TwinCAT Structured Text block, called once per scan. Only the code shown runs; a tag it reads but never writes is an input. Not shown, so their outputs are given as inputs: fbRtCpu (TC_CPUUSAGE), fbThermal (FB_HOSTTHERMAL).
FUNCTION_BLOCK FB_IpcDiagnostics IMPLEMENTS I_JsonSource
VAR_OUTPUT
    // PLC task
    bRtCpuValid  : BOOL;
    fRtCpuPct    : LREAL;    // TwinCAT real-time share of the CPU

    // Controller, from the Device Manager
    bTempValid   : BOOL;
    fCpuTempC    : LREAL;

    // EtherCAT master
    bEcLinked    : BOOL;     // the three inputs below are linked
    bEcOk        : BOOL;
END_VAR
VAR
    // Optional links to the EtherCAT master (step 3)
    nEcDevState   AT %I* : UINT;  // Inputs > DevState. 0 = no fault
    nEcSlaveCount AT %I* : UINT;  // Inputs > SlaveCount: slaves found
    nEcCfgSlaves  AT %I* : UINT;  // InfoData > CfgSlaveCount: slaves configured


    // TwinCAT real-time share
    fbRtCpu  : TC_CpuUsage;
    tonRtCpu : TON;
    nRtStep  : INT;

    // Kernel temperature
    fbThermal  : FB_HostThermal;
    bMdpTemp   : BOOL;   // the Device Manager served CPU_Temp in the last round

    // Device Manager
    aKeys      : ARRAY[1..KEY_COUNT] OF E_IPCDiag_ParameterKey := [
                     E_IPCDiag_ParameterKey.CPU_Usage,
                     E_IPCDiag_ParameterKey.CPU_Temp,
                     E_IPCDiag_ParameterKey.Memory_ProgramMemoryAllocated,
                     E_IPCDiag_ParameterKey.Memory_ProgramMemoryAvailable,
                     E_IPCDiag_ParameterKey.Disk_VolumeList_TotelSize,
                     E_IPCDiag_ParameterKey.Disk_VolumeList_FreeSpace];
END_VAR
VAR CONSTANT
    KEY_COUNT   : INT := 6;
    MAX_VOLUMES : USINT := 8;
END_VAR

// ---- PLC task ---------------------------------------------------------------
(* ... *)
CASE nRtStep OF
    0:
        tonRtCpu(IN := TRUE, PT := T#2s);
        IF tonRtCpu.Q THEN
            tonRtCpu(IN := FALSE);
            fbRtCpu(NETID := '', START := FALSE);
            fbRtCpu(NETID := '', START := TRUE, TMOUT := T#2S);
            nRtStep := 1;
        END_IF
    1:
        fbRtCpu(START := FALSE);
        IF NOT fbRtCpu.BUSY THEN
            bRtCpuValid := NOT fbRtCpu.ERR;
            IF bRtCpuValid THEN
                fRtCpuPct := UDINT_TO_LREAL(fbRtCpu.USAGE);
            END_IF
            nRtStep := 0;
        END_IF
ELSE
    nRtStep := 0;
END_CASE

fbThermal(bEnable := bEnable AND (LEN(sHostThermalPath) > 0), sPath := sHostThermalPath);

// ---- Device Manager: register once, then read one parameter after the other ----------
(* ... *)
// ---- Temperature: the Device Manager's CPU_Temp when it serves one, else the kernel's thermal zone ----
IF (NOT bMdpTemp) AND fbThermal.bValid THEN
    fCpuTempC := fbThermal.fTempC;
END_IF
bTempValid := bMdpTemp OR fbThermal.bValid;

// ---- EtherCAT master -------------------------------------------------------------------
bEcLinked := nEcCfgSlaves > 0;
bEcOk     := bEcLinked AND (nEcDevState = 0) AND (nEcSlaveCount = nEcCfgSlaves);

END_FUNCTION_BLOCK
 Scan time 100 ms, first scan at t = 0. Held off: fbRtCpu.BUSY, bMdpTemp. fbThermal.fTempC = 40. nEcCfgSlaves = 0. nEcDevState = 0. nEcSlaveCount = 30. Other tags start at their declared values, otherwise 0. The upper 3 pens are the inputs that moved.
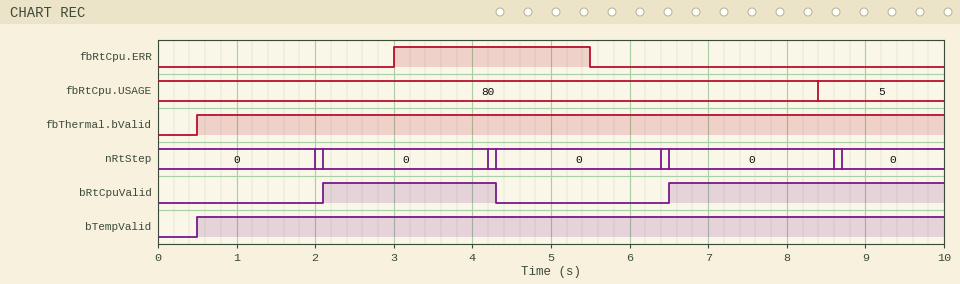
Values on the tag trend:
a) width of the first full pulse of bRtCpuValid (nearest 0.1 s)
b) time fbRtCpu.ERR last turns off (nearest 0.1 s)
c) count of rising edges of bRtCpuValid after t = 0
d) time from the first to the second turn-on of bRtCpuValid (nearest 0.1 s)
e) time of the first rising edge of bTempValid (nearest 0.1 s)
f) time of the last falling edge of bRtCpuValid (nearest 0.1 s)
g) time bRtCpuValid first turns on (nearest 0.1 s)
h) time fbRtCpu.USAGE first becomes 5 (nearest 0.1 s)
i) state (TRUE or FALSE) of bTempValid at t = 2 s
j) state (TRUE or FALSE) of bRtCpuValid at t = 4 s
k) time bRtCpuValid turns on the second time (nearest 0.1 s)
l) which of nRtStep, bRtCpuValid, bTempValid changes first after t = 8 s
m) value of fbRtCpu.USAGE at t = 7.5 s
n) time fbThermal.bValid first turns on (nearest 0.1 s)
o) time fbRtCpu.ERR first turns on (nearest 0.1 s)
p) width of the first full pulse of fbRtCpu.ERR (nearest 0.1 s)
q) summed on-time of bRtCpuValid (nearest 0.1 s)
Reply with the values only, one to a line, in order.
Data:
2.2 s
5.5 s
2
4.4 s
0.5 s
4.3 s
2.1 s
8.4 s
TRUE
TRUE
6.5 s
nRtStep
80
0.5 s
3.0 s
2.5 s
5.7 s
